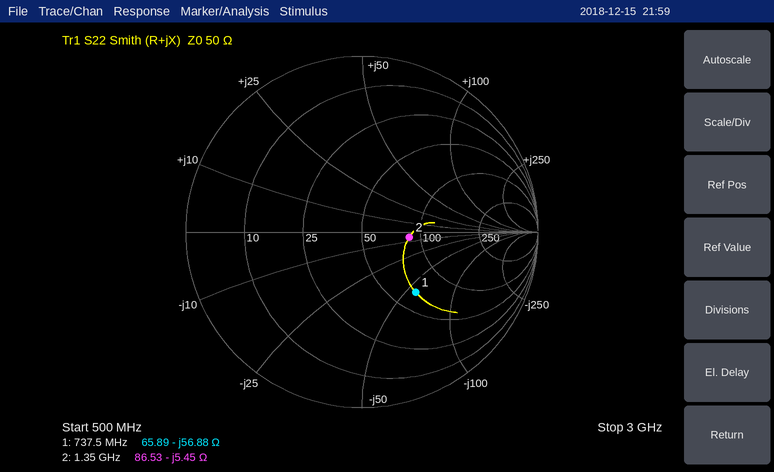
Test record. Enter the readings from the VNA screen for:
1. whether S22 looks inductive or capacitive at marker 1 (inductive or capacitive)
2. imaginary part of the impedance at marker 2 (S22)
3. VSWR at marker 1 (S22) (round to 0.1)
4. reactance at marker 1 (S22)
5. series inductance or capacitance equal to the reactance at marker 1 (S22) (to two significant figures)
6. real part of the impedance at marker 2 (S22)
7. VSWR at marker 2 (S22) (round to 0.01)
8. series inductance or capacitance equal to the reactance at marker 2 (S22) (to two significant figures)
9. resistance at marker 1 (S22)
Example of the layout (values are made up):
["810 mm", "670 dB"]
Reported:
["capacitive", "-5.45 Ω", "2.7", "-56.88 Ω", "3.8 pF", "86.53 Ω", "1.74", "22 pF", "65.89 Ω"]
